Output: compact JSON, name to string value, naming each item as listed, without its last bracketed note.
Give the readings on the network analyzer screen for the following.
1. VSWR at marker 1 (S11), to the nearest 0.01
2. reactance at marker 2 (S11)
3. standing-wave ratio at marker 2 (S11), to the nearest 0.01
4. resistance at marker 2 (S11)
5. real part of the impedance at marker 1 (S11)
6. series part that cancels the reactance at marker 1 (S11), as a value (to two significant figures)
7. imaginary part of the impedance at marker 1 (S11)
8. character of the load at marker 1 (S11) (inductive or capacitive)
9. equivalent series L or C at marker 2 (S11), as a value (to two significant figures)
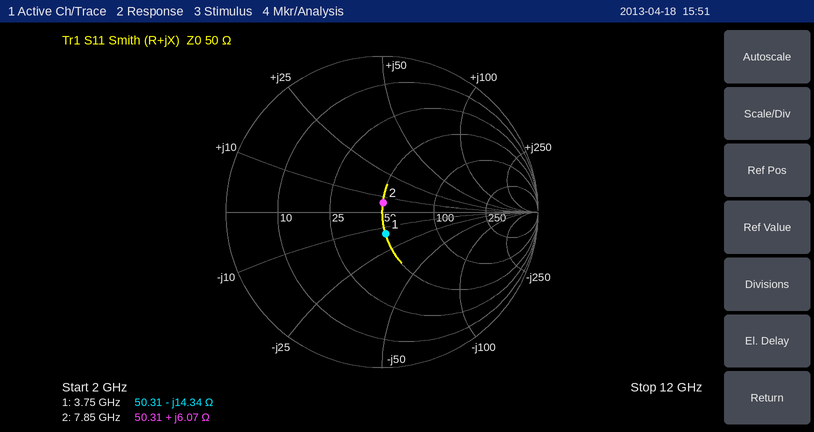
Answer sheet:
{"VSWR at marker 1 (S11), to the nearest 0.01": "1.33", "reactance at marker 2": "+6.07 Ω", "standing-wave ratio at marker 2 (S11), to the nearest 0.01": "1.13", "resistance at marker 2": "50.31 Ω", "real part of the impedance at marker 1": "50.31 Ω", "series part that cancels the reactance at marker 1 (S11), as a value": "610 pH", "imaginary part of the impedance at marker 1": "-14.34 Ω", "character of the load at marker 1 (S11)": "capacitive", "equivalent series L or C at marker 2 (S11), as a value": "120 pH"}
